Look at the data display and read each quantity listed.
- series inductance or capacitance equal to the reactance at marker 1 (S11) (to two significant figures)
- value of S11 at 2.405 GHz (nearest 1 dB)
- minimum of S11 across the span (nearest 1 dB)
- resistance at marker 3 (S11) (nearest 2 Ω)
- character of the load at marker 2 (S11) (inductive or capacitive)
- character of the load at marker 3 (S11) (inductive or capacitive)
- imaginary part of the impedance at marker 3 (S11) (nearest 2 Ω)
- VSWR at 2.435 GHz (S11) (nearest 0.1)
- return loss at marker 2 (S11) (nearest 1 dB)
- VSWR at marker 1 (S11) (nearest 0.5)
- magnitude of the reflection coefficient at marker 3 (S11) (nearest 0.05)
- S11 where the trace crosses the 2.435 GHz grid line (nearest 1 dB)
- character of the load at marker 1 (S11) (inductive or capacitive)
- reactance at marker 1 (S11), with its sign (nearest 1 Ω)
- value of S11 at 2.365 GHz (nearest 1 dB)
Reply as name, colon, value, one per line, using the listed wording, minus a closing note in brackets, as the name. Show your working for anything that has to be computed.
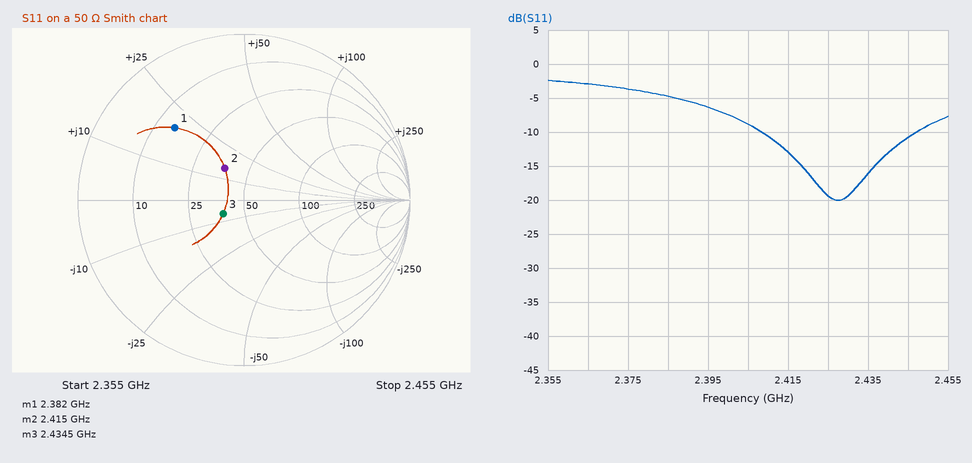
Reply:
series inductance or capacitance equal to the reactance at marker 1 (S11): L = 20 Ω/(2π × 2.382 GHz) ≈ 1.3 nH
value of S11 at 2.405 GHz: -9 dB
minimum of S11 across the span: -20 dB
resistance at marker 3 (S11): 38 Ω
character of the load at marker 2 (S11): inductive
character of the load at marker 3 (S11): capacitive
imaginary part of the impedance at marker 3 (S11): -6 Ω
VSWR at 2.435 GHz (S11): |Γ| = 10^(-16/20) = 0.1585; VSWR = (1 + 0.1585)/(1 − 0.1585) ≈ 1.4
return loss at marker 2 (S11): 13 dB
VSWR at marker 1 (S11): 4.0
magnitude of the reflection coefficient at marker 3 (S11): 0.15
S11 where the trace crosses the 2.435 GHz grid line: -16 dB
character of the load at marker 1 (S11): inductive
reactance at marker 1 (S11), with its sign: +20 Ω
value of S11 at 2.365 GHz: -3 dB
